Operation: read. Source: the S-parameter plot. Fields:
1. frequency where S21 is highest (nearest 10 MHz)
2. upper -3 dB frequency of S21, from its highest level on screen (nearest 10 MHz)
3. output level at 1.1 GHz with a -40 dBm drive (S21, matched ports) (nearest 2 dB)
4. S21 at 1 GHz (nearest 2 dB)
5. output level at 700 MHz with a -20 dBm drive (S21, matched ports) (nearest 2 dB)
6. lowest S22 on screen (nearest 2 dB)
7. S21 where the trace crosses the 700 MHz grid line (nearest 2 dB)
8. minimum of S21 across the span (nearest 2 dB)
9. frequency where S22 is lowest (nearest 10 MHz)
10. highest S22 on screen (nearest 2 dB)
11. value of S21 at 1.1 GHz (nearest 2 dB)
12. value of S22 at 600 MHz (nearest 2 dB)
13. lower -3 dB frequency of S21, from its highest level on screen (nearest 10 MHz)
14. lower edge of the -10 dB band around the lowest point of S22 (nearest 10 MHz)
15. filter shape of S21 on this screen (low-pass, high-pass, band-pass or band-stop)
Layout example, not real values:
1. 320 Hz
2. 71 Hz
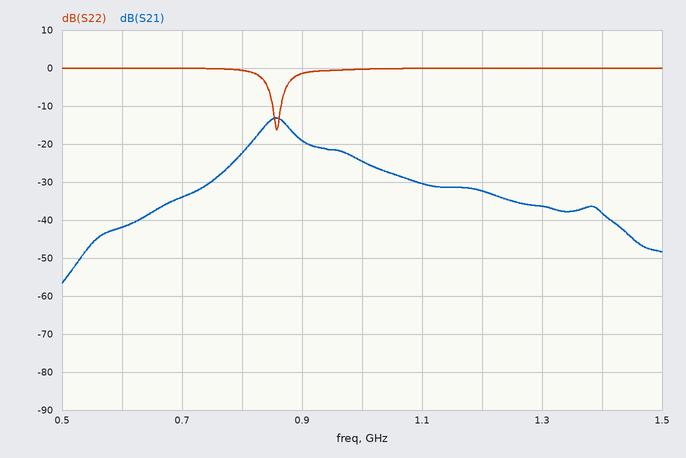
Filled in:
1. 860 MHz
2. 880 MHz
3. -70 dBm
4. -24 dB
5. -54 dBm
6. -16 dB
7. -34 dB
8. -56 dB
9. 860 MHz
10. 0 dB
11. -30 dB
12. 0 dB
13. 830 MHz
14. 850 MHz
15. band-pass
